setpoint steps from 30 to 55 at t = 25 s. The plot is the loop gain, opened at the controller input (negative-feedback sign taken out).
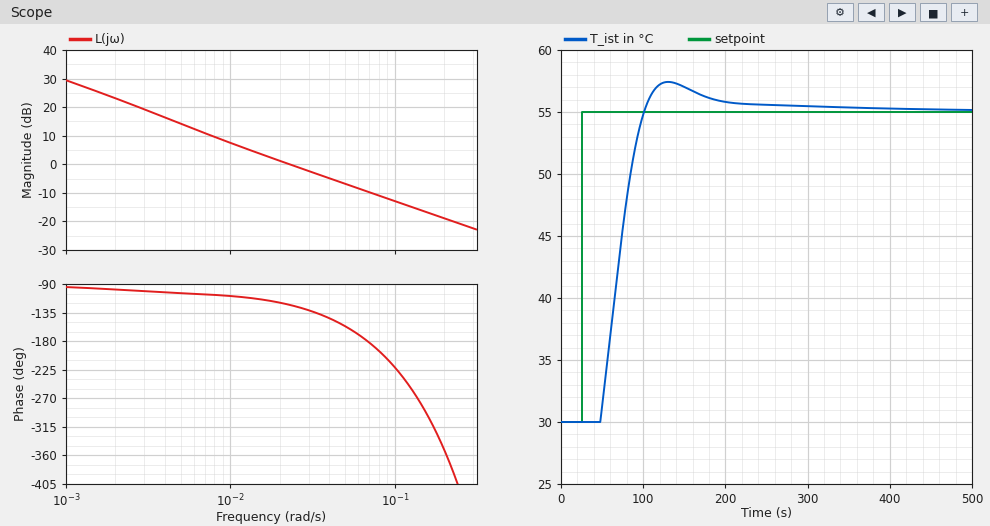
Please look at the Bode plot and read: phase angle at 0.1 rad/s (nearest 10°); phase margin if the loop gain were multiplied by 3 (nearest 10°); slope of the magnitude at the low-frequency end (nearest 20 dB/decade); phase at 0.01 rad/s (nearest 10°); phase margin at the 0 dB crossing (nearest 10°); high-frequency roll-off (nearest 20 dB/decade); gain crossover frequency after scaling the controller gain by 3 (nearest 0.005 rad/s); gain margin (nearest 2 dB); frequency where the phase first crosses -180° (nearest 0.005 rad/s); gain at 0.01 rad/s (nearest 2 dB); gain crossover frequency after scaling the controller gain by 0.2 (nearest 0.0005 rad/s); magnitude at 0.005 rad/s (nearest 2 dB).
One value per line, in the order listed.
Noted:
-220°
0°
-20 dB/decade
-110°
60°
-20 dB/decade
0.070 rad/s
10 dB
0.070 rad/s
8 dB
0.0050 rad/s
14 dB
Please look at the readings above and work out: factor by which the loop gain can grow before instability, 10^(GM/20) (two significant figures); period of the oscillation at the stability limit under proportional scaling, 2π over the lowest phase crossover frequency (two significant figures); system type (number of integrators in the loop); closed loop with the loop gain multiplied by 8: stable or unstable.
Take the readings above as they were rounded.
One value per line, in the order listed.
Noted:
3.2
90 s
1
unstable
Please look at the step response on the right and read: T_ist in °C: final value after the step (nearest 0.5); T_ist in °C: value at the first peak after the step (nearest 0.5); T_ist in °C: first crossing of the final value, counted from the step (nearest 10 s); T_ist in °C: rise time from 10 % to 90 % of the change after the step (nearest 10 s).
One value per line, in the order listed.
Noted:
55.0
57.5
80 s
40 s
